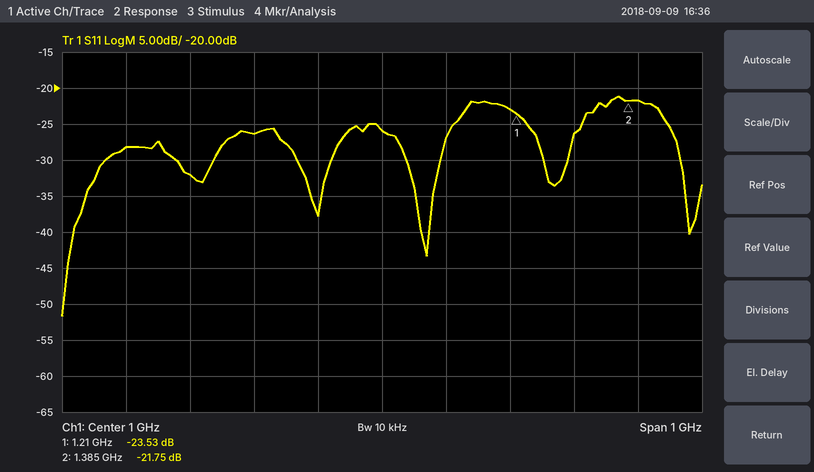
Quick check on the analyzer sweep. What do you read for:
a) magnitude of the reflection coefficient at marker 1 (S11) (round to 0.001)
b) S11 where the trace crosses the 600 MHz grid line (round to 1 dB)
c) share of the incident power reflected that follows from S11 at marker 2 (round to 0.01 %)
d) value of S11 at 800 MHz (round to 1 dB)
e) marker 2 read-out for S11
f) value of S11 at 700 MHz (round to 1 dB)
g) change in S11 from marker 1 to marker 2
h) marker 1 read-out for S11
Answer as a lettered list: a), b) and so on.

a) 0.067
b) -28 dB
c) 0.67 %
d) -26 dB
e) -21.75 dB
f) -32 dB
g) 1.78 dB
h) -23.53 dB
